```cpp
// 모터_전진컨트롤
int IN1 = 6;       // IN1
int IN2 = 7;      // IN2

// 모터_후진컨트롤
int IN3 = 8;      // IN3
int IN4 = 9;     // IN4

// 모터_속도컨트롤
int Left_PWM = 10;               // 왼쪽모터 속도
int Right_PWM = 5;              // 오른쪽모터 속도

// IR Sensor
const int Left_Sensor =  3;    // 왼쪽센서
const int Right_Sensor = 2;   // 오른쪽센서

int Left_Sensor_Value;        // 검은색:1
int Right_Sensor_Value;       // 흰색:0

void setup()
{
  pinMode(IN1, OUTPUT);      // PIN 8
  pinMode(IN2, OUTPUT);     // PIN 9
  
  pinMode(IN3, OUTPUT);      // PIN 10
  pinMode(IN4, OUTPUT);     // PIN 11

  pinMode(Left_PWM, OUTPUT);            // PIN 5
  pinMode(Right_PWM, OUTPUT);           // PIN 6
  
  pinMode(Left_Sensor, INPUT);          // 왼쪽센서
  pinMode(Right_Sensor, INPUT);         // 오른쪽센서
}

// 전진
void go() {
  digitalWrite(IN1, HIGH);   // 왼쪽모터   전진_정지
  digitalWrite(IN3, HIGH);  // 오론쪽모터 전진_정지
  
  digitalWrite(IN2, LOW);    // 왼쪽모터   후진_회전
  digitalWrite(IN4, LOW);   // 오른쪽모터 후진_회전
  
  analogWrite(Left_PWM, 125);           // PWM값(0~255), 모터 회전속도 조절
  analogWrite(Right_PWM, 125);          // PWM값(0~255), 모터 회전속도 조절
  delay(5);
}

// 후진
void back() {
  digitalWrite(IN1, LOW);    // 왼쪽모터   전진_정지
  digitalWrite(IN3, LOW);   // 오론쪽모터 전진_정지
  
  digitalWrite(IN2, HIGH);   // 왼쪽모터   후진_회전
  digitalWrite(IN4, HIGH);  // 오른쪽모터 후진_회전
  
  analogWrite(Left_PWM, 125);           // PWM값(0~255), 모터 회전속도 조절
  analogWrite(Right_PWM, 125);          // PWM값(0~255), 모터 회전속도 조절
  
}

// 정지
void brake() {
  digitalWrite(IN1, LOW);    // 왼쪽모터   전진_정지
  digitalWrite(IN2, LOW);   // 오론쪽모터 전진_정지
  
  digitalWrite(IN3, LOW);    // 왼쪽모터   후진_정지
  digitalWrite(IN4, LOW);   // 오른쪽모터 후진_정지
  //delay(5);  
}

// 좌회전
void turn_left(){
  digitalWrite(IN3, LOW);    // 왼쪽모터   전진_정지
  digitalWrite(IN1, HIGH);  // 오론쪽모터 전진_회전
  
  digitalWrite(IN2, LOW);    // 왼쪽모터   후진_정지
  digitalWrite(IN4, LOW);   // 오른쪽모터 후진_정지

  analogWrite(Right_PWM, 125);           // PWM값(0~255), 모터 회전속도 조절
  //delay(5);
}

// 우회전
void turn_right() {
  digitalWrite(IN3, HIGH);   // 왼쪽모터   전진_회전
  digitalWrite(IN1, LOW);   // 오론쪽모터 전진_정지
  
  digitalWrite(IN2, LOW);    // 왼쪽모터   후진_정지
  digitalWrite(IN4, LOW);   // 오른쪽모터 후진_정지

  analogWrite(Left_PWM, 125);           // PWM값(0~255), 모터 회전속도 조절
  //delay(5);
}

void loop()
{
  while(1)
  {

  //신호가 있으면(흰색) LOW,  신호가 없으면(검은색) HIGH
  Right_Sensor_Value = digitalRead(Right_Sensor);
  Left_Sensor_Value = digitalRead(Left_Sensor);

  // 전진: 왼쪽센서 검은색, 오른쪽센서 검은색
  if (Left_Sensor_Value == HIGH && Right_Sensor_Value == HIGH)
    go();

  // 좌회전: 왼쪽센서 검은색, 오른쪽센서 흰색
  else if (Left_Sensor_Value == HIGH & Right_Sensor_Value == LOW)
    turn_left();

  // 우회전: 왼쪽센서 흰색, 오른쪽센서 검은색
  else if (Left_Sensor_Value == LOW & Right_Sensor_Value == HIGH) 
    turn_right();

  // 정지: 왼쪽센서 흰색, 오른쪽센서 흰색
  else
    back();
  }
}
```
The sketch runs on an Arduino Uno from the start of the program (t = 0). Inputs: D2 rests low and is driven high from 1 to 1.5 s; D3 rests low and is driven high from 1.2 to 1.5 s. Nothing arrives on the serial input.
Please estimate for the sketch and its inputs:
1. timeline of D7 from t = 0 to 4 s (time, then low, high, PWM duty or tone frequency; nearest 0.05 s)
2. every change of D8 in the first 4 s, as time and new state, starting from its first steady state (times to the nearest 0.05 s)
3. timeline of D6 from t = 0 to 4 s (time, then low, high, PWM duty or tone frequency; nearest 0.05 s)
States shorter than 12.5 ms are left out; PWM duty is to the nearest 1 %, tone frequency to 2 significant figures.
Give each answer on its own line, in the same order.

0 s high; 1 s low; 1.5 s high
0 s low; 1 s high; 1.5 s low
0 s low; 1.2 s high; 1.5 s low
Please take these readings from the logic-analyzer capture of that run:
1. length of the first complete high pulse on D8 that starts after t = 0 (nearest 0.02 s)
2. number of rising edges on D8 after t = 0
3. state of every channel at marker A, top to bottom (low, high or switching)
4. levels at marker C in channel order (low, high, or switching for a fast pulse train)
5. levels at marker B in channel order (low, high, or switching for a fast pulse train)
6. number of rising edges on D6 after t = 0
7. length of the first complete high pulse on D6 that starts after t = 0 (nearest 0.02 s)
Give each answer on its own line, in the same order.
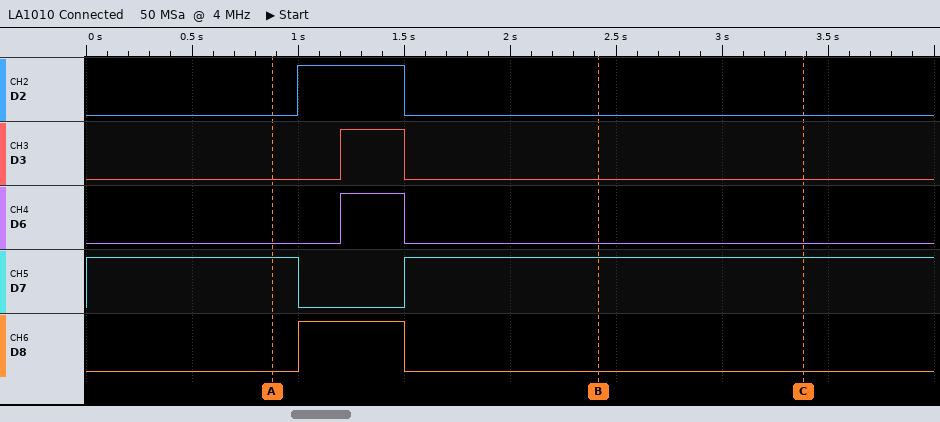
0.50 s
1
D2 low, D3 low, D6 low, D7 high, D8 low
D2 low, D3 low, D6 low, D7 high, D8 low
D2 low, D3 low, D6 low, D7 high, D8 low
1
0.30 s
